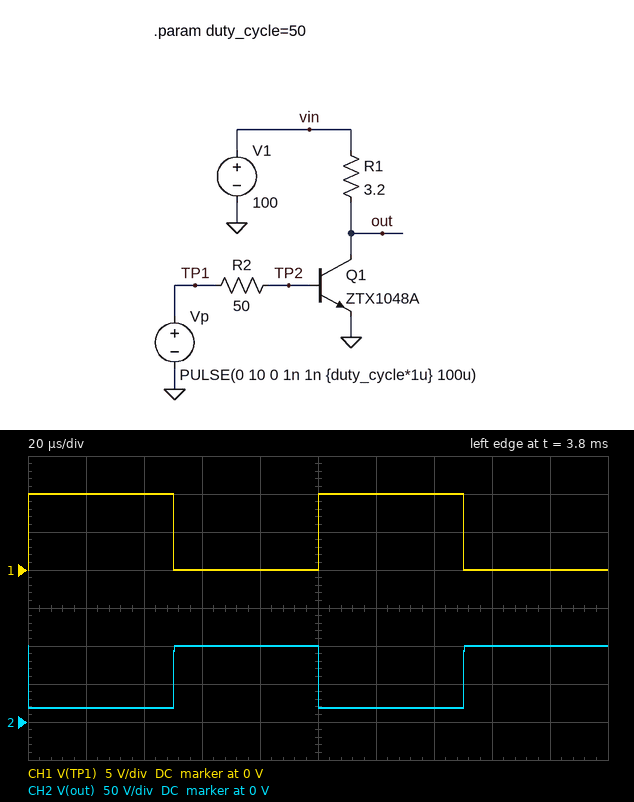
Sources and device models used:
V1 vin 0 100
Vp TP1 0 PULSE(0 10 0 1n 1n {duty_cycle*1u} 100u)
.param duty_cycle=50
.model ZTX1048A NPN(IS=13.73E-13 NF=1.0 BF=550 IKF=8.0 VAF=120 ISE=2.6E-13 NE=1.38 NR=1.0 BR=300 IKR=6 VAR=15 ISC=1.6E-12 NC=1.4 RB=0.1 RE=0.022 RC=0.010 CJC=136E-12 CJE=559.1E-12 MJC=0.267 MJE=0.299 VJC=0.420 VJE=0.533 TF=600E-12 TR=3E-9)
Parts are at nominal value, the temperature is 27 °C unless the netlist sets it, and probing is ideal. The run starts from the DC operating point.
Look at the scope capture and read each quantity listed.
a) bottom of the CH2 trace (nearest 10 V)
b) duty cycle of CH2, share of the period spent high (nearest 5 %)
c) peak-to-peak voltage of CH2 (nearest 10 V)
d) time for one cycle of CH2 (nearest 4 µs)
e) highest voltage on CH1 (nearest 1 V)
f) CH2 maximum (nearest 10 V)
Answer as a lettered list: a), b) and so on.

a) 20 V
b) 50 %
c) 80 V
d) 100 µs
e) 10 V
f) 100 V
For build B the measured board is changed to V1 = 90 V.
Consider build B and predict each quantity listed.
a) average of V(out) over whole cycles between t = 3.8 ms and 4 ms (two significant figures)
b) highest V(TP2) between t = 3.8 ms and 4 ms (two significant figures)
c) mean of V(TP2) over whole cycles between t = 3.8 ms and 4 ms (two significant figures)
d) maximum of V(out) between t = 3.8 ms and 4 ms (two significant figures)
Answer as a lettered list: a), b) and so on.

a) 51 V
b) 1.4 V
c) 690 mV
d) 90 V
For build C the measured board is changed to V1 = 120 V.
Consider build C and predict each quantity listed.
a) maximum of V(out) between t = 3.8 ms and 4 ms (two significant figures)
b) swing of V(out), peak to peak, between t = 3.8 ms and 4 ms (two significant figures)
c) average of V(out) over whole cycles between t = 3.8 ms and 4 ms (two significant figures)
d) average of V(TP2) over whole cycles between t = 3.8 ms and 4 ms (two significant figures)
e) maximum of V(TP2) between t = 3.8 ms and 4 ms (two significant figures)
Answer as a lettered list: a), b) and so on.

a) 120 V
b) 89 V
c) 75 V
d) 730 mV
e) 1.5 V
